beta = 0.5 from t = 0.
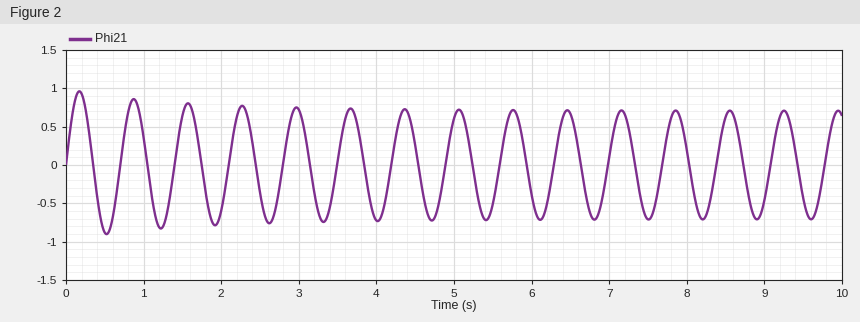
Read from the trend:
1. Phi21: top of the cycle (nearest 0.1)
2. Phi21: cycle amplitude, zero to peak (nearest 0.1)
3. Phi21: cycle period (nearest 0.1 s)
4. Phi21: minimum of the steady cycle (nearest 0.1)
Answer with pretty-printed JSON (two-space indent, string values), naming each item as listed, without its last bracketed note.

{
  "Phi21: top of the cycle": "0.7",
  "Phi21: cycle amplitude, zero to peak": "0.7",
  "Phi21: cycle period": "0.7 s",
  "Phi21: minimum of the steady cycle": "-0.7"
}
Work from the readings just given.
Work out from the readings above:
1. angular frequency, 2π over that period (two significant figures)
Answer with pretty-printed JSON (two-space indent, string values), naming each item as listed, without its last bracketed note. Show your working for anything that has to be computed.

{
  "angular frequency, 2π over that period": "2π / 0.7 = 9.0 rad/s"
}
